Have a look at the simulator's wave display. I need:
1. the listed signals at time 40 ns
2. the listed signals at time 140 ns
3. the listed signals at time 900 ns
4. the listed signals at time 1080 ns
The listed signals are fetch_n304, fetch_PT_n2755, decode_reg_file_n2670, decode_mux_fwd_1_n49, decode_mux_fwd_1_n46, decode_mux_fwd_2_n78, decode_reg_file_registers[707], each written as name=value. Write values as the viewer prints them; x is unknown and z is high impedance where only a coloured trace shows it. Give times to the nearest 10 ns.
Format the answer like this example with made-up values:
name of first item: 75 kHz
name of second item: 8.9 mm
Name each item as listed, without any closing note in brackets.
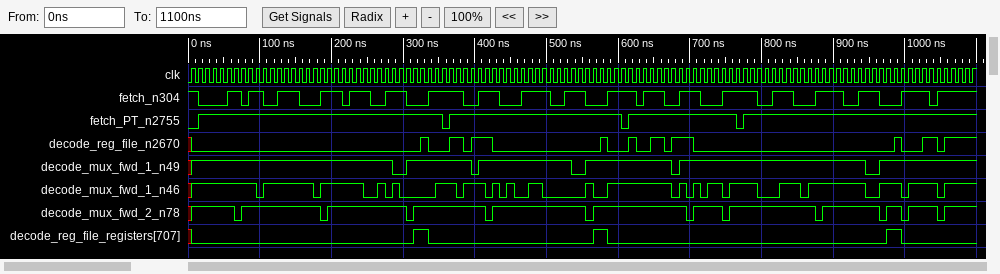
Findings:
the listed signals at time 40 ns: fetch_n304=0, fetch_PT_n2755=1, decode_reg_file_n2670=0, decode_mux_fwd_1_n49=1, decode_mux_fwd_1_n46=1, decode_mux_fwd_2_n78=1, decode_reg_file_registers[707]=0
the listed signals at time 140 ns: fetch_n304=1, fetch_PT_n2755=1, decode_reg_file_n2670=0, decode_mux_fwd_1_n49=1, decode_mux_fwd_1_n46=1, decode_mux_fwd_2_n78=1, decode_reg_file_registers[707]=0
the listed signals at time 900 ns: fetch_n304=1, fetch_PT_n2755=1, decode_reg_file_n2670=0, decode_mux_fwd_1_n49=1, decode_mux_fwd_1_n46=1, decode_mux_fwd_2_n78=1, decode_reg_file_registers[707]=0
the listed signals at time 1080 ns: fetch_n304=1, fetch_PT_n2755=1, decode_reg_file_n2670=1, decode_mux_fwd_1_n49=1, decode_mux_fwd_1_n46=1, decode_mux_fwd_2_n78=1, decode_reg_file_registers[707]=0
